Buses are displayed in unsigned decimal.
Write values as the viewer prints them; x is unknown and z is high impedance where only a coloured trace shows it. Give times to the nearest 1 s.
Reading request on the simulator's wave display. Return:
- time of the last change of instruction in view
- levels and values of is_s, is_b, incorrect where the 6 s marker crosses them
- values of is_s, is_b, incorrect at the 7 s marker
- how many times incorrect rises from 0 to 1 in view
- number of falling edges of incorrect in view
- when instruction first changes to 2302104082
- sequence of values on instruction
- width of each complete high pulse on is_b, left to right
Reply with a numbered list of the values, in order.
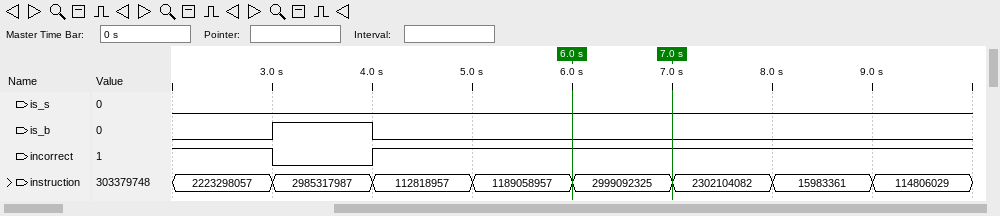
1. 9 s
2. is_s=0, is_b=0, incorrect=1
3. is_s=0, is_b=0, incorrect=1
4. 1
5. 1
6. 7 s
7. 2223298057, 2985317987, 112818957, 1189058957, 2999092325, 2302104082, 15983361, 114806029
8. 1 s
